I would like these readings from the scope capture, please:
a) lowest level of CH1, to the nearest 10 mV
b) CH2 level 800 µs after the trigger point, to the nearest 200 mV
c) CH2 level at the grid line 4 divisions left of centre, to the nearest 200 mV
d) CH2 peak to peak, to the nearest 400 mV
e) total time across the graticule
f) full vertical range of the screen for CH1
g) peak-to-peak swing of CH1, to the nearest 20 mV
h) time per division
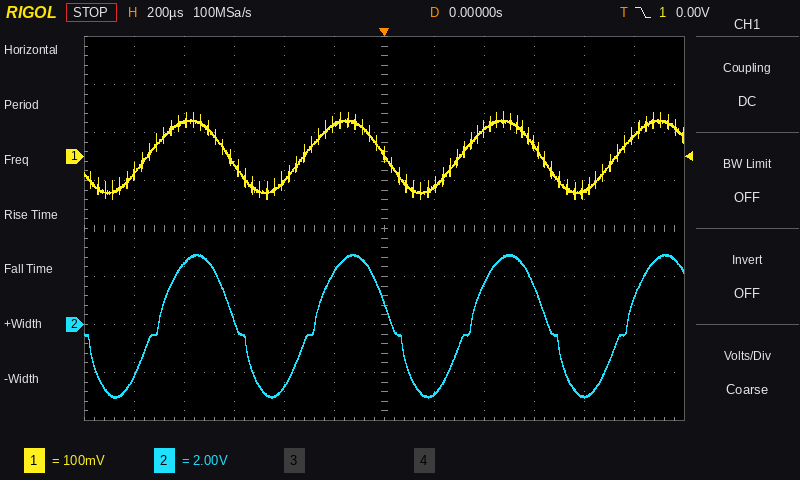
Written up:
-90 mV
-3.0 V
2.6 V
6.0 V
2.4 ms
800 mV
180 mV
200 µs
